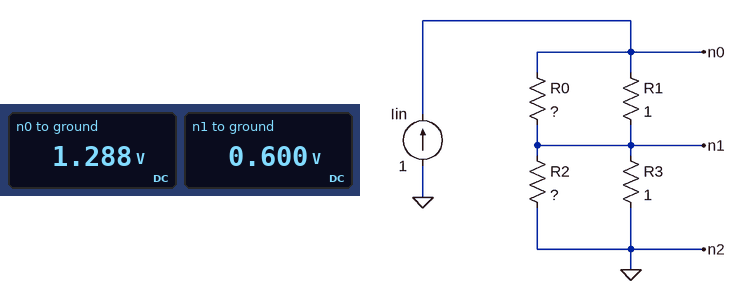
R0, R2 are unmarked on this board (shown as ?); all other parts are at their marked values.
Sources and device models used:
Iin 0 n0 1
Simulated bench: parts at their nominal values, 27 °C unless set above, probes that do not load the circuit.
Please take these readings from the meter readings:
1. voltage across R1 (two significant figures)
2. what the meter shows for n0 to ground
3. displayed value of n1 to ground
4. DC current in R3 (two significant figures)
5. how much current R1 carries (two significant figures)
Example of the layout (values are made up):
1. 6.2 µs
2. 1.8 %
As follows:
1. 690 mV
2. 1.288 V
3. 0.600 V
4. 600 mA
5. 690 mA
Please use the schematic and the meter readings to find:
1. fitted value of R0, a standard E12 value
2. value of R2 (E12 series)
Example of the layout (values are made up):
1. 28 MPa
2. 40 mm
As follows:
1. 2.2 Ω
2. 1.5 Ω
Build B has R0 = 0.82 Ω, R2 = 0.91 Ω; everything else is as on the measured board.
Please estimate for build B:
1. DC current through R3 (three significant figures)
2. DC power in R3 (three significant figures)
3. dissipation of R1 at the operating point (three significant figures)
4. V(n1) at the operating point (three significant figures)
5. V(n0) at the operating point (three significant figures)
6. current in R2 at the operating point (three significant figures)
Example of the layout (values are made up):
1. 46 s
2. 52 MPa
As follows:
1. 476 mA
2. 227 mW
3. 203 mW
4. 476 mV
5. 927 mV
6. 524 mA
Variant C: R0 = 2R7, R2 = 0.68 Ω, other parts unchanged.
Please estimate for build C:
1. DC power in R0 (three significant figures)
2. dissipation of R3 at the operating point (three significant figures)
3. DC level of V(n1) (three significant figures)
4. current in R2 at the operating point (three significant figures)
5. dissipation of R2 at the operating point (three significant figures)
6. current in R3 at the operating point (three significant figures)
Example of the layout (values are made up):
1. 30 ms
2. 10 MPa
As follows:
1. 197 mW
2. 164 mW
3. 405 mV
4. 595 mA
5. 241 mW
6. 405 mA
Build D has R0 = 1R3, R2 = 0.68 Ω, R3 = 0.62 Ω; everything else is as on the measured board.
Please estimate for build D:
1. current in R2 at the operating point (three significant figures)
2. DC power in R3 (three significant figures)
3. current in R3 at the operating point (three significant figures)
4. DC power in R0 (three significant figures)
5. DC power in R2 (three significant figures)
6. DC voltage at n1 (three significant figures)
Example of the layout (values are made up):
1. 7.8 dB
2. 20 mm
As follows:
1. 477 mA
2. 170 mW
3. 523 mA
4. 246 mW
5. 155 mW
6. 324 mV
